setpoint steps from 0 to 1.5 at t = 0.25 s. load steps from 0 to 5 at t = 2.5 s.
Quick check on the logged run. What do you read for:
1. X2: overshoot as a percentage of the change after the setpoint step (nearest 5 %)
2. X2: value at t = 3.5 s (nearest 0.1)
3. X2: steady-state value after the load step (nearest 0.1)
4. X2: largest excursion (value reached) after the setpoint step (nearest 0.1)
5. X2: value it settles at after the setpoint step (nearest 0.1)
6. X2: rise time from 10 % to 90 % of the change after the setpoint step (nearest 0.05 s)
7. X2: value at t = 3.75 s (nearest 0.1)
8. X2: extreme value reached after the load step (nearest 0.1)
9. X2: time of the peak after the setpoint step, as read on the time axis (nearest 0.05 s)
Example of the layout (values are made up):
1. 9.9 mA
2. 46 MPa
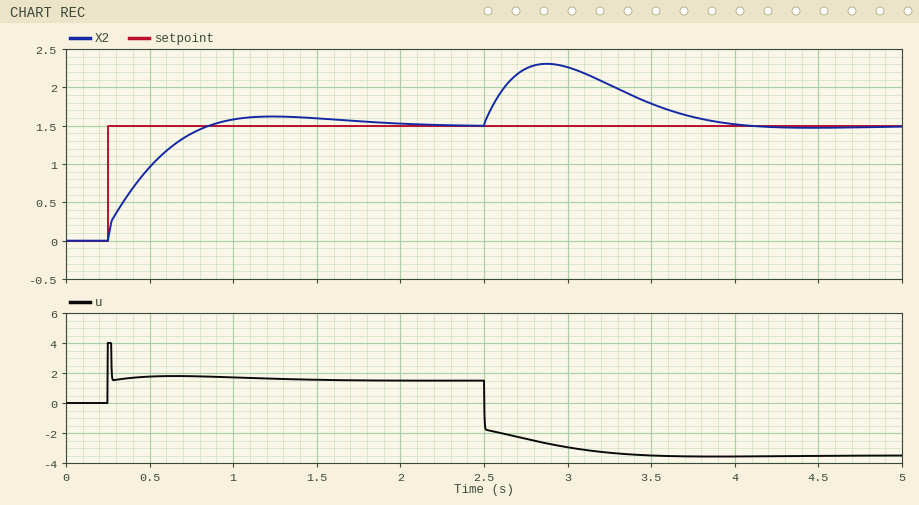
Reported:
1. 10 %
2. 1.8
3. 1.5
4. 1.6
5. 1.5
6. 0.45 s
7. 1.6
8. 2.3
9. 1.25 s
